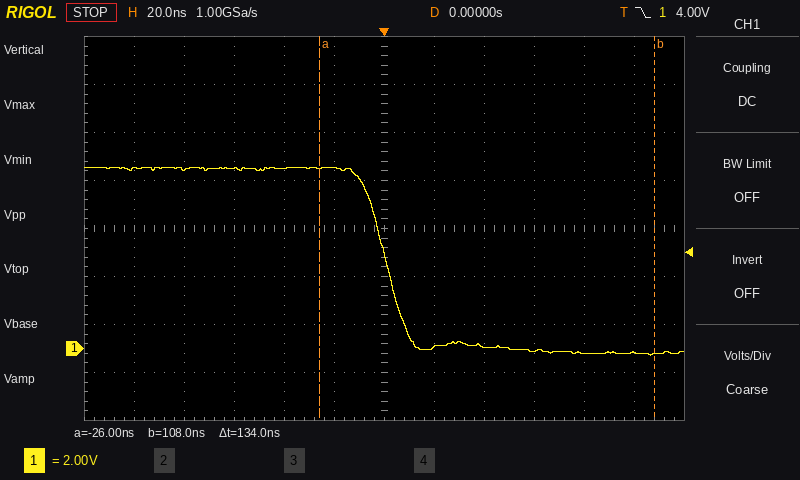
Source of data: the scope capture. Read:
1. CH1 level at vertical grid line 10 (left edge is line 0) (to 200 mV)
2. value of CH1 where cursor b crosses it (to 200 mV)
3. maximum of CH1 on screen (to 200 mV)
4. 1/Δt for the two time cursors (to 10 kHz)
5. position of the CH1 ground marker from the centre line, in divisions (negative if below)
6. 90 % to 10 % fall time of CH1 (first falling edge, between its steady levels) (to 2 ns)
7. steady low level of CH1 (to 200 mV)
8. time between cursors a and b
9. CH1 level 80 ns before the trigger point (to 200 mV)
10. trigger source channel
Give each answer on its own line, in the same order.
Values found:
-200 mV
-200 mV
7.6 V
7.46 MHz
-2.5 div
18 ns
-200 mV
134 ns
7.4 V
CH1
